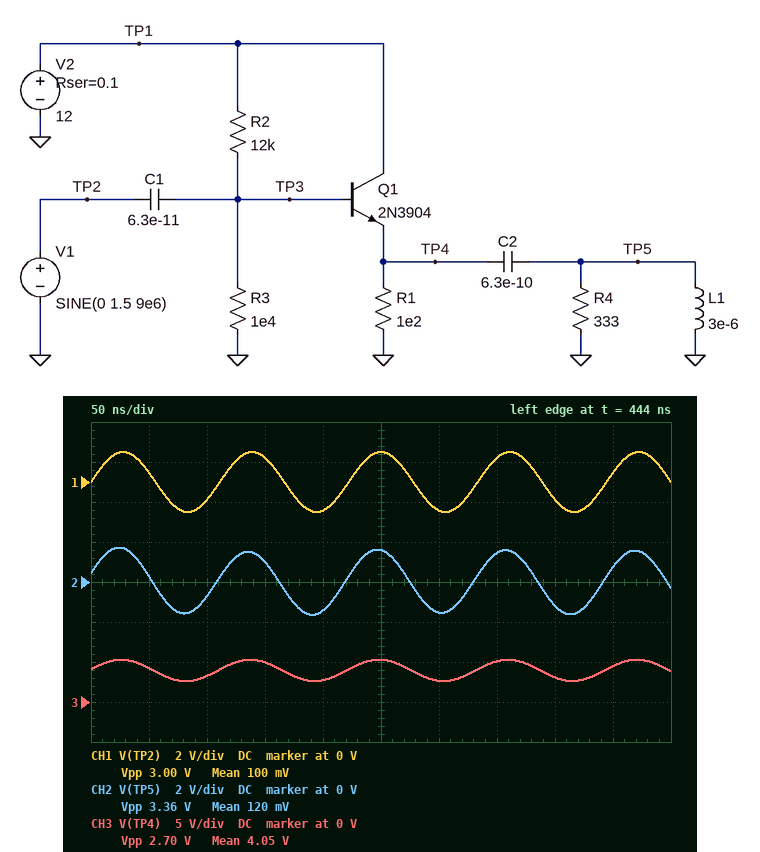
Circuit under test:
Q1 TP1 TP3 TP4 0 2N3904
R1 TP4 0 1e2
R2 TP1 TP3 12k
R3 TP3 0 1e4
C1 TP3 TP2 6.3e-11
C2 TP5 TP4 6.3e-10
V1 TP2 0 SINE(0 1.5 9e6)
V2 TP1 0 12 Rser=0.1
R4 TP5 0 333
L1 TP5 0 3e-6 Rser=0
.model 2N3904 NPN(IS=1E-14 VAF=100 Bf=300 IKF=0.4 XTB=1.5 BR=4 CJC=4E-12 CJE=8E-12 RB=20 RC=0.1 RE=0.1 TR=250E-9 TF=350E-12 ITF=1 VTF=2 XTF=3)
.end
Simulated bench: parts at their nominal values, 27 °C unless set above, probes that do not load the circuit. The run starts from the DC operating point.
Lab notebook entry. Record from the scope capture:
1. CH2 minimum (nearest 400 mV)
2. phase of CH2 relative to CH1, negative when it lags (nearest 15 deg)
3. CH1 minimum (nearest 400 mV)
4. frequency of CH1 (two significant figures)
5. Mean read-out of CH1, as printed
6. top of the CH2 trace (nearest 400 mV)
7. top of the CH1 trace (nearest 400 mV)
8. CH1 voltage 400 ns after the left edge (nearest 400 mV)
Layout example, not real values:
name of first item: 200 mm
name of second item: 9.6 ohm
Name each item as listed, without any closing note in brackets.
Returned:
CH2 minimum: -1.6 V
phase of CH2 relative to CH1, negative when it lags: 15 deg
CH1 minimum: -1.6 V
frequency of CH1: 9.0 MHz
Mean read-out of CH1, as printed: 100 mV
top of the CH2 trace: 1.6 V
top of the CH1 trace: 1.6 V
CH1 voltage 400 ns after the left edge: -800 mV
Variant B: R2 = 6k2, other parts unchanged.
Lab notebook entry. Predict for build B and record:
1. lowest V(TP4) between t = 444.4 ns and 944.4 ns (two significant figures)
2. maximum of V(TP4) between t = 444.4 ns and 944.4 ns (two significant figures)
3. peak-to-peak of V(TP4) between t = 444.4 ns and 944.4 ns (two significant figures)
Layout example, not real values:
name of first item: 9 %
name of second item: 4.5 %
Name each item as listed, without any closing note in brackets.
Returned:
lowest V(TP4) between t = 444.4 ns and 944.4 ns: 4.5 V
maximum of V(TP4) between t = 444.4 ns and 944.4 ns: 7.2 V
peak-to-peak of V(TP4) between t = 444.4 ns and 944.4 ns: 2.7 V
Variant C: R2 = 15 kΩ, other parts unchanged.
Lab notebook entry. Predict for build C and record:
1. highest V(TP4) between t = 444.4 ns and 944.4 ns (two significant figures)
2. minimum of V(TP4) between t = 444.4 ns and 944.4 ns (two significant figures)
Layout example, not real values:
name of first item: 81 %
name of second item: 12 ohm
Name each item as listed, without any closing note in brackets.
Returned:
highest V(TP4) between t = 444.4 ns and 944.4 ns: 4.7 V
minimum of V(TP4) between t = 444.4 ns and 944.4 ns: 2.0 V
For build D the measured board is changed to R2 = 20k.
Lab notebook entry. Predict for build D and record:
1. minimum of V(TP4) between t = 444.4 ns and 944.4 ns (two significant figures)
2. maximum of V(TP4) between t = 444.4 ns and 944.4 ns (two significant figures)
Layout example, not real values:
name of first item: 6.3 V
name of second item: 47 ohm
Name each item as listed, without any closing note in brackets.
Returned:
minimum of V(TP4) between t = 444.4 ns and 944.4 ns: 1.3 V
maximum of V(TP4) between t = 444.4 ns and 944.4 ns: 4.0 V
